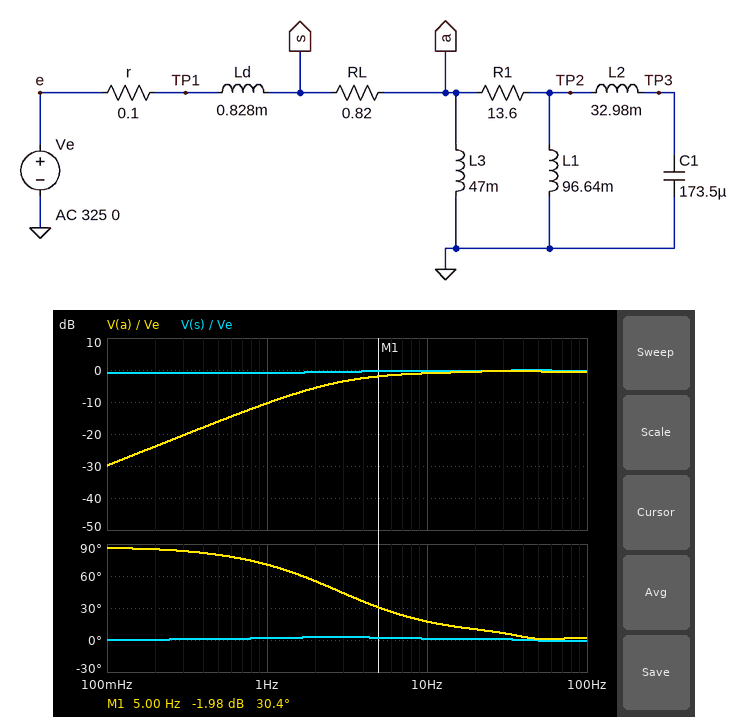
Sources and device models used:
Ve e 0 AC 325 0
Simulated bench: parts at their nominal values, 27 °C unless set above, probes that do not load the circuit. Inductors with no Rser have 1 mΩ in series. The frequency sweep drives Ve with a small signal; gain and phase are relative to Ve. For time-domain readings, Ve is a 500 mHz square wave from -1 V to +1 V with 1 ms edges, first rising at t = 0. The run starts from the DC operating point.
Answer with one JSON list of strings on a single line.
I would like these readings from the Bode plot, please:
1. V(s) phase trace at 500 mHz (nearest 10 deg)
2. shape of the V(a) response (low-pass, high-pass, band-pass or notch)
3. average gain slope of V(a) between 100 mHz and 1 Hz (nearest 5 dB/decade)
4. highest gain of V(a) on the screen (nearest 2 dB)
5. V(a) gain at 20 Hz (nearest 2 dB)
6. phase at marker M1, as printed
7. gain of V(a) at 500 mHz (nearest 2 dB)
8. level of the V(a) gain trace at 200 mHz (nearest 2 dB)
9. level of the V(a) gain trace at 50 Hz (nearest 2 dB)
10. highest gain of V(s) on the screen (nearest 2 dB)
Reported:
["0 deg", "high-pass", "20 dB/decade", "0 dB", "0 dB", "30.4 deg", "-16 dB", "-24 dB", "0 dB", "0 dB"]
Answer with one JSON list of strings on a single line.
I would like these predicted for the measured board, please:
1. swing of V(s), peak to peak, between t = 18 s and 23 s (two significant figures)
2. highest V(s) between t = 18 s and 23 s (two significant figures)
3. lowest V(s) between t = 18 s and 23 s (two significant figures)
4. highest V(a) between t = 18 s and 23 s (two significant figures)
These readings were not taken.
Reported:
["2.1 V", "1.1 V", "-1.1 V", "1.9 V"]
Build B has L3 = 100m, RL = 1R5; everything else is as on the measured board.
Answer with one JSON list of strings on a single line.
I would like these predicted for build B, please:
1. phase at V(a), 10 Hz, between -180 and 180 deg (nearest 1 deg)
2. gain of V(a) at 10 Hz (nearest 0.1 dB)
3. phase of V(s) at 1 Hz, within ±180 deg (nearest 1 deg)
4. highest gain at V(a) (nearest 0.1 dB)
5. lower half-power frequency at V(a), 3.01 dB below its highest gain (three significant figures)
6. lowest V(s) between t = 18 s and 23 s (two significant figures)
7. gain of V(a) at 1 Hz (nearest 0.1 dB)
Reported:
["15 deg", "-1.2 dB", "1 deg", "-0.1 dB", "2.94 Hz", "-1.0 V", "-8.9 dB"]
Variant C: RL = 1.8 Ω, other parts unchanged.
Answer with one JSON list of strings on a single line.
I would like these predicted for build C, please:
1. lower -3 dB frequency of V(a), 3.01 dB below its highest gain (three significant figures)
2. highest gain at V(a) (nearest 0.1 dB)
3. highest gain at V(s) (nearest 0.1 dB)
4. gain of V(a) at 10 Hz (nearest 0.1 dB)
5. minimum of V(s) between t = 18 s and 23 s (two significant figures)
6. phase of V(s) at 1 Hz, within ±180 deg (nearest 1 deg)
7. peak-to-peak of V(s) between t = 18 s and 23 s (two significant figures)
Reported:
["7.46 Hz", "-0.3 dB", "-0.1 dB", "-2.5 dB", "-1.0 V", "0 deg", "2.0 V"]
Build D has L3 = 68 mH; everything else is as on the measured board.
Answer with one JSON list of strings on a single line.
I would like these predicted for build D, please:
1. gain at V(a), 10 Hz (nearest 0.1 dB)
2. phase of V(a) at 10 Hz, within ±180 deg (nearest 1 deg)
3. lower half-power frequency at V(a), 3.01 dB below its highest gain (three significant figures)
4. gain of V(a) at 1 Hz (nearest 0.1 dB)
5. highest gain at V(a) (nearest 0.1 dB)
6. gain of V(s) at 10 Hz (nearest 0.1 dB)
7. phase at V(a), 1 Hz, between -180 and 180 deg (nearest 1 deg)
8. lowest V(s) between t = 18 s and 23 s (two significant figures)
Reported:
["-0.8 dB", "13 deg", "2.31 Hz", "-7.7 dB", "-0.1 dB", "-0.2 dB", "63 deg", "-1.1 V"]
